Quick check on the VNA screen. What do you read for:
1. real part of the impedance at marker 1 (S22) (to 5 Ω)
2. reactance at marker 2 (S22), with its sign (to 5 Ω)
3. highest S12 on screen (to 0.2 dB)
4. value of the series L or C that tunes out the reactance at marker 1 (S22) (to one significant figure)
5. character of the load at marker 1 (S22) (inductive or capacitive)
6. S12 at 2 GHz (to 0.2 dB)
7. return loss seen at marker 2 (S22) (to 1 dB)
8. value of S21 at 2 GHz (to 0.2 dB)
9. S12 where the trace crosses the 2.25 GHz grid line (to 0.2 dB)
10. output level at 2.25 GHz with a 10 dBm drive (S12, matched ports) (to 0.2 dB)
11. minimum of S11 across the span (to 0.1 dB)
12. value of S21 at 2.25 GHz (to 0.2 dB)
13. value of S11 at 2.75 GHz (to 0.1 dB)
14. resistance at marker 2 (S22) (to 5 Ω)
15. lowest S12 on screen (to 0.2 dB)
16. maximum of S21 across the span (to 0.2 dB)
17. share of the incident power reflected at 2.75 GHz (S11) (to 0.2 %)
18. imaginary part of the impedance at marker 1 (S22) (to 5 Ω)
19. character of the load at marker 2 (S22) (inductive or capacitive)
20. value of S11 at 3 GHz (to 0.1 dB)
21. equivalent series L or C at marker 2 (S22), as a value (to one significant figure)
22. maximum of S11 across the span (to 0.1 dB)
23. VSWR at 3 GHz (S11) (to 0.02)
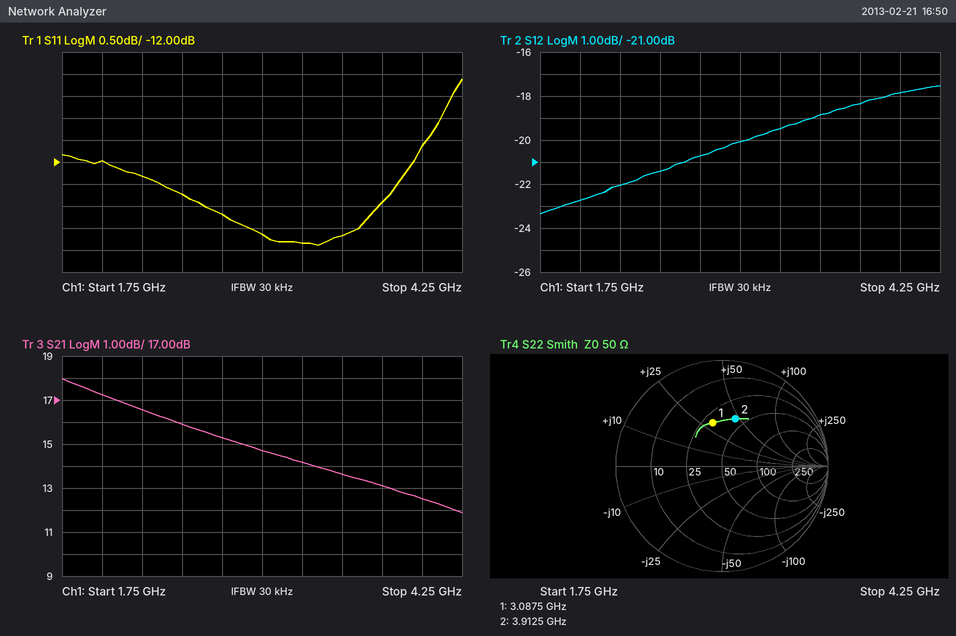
30 Ω
+45 Ω
-17.6 dB
2 pF
inductive
-22.8 dB
7 dB
17.2 dB
-22.0 dB
-12.0 dBm
-13.9 dB
16.6 dB
-13.2 dB
40 Ω
-23.4 dB
18.0 dB
4.8 %
+30 Ω
inductive
-13.6 dB
2 nH
-10.1 dB
1.52
